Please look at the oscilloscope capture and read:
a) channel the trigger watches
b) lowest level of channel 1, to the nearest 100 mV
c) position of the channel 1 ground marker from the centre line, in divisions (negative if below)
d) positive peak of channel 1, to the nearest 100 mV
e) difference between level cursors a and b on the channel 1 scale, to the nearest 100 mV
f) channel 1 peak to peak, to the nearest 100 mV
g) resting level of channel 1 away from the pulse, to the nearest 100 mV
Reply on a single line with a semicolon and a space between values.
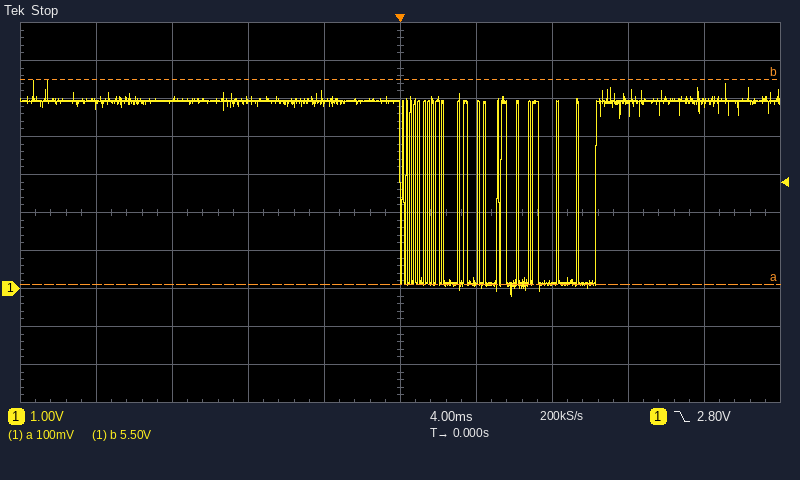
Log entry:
channel 1; -200 mV; -2.0 div; 5.5 V; 5.4 V; 5.7 V; 4.9 V
